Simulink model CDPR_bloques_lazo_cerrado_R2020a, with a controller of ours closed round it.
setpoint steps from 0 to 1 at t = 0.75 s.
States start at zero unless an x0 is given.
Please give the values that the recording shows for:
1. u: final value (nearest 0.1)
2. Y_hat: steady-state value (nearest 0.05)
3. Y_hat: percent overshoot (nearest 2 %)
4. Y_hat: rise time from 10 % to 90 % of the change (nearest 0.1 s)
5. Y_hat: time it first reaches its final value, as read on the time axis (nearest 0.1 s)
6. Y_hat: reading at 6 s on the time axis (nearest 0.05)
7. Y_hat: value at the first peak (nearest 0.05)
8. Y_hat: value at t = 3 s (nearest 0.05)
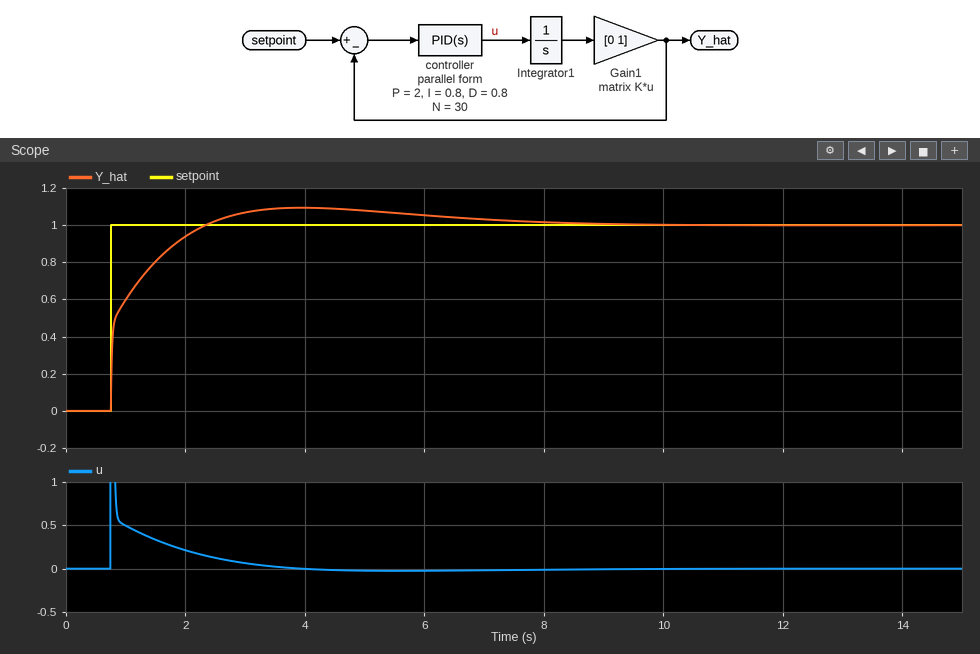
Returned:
0.0
1.00
10 %
1.1 s
2.3 s
1.05
1.10
1.05
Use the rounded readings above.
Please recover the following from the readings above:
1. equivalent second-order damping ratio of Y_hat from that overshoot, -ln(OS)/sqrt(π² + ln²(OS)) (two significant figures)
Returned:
0.59
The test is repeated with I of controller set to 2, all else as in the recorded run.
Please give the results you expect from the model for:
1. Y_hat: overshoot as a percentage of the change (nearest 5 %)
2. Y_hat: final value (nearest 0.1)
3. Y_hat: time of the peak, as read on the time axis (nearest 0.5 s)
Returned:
15 %
1.0
3.0 s
